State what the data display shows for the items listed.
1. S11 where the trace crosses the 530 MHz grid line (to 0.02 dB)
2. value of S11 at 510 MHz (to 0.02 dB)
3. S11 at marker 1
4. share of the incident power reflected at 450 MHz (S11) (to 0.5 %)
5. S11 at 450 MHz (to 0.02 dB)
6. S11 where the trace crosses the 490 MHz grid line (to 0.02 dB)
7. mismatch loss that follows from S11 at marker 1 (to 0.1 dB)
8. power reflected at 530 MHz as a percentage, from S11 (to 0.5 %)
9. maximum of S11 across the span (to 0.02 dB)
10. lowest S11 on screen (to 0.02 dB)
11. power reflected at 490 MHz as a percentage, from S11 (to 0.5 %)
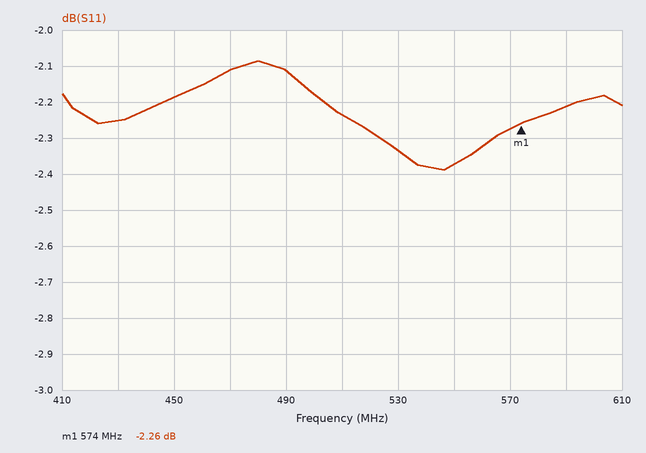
-2.34 dB
-2.24 dB
-2.26 dB
60.5 %
-2.18 dB
-2.12 dB
3.9 dB
58.5 %
-2.08 dB
-2.38 dB
61.5 %
